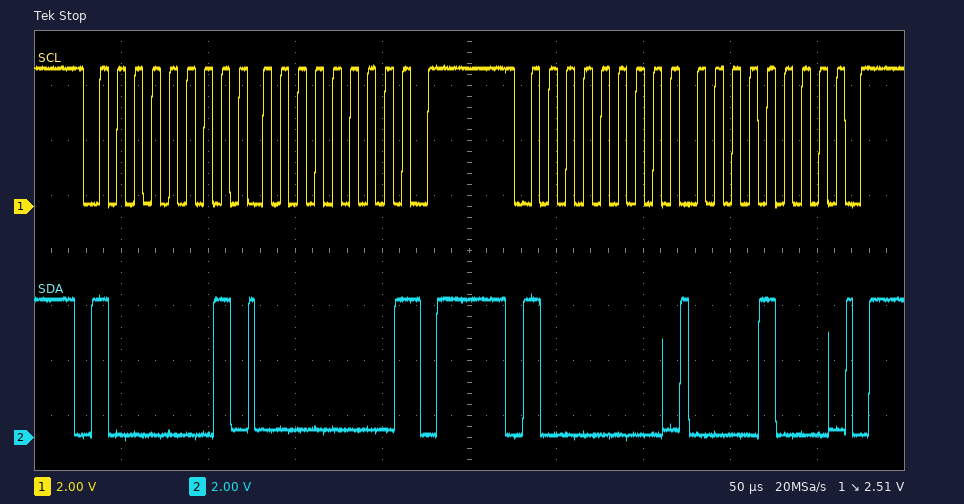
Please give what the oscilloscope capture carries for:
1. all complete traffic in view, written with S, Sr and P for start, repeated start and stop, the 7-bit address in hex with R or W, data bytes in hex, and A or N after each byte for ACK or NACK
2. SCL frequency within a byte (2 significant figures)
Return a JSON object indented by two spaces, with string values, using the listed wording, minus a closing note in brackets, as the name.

{
  "all complete traffic in view, written with S, Sr and P for start, repeated start and stop, the 7-bit address in hex with R or W, data bytes in hex, and A or N after each byte for ACK or NACK": "S 40R A 00 N P S 40W A 08 A P",
  "SCL frequency within a byte": "100 kHz"
}
